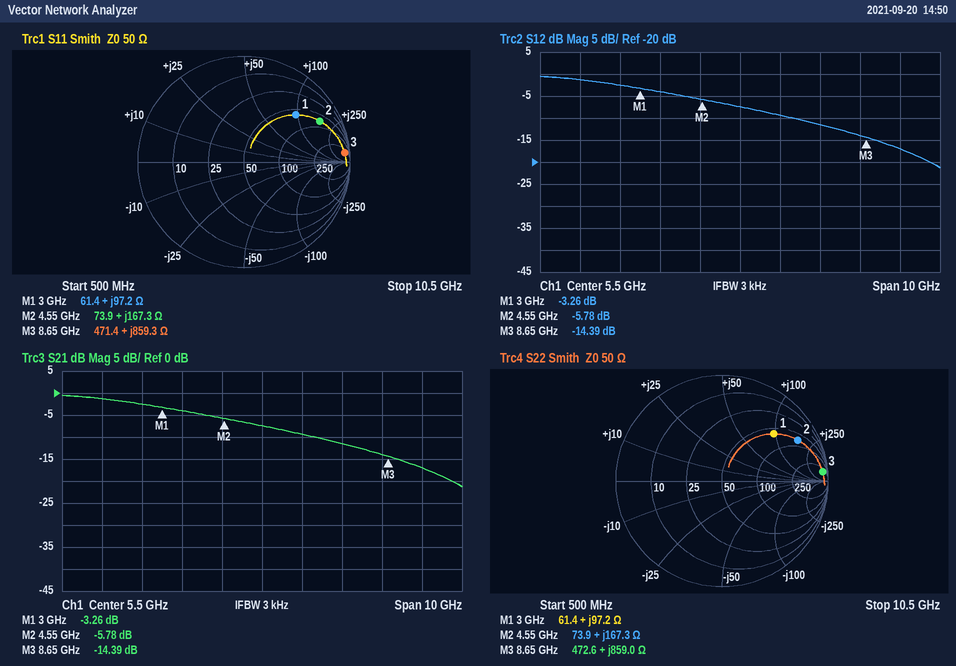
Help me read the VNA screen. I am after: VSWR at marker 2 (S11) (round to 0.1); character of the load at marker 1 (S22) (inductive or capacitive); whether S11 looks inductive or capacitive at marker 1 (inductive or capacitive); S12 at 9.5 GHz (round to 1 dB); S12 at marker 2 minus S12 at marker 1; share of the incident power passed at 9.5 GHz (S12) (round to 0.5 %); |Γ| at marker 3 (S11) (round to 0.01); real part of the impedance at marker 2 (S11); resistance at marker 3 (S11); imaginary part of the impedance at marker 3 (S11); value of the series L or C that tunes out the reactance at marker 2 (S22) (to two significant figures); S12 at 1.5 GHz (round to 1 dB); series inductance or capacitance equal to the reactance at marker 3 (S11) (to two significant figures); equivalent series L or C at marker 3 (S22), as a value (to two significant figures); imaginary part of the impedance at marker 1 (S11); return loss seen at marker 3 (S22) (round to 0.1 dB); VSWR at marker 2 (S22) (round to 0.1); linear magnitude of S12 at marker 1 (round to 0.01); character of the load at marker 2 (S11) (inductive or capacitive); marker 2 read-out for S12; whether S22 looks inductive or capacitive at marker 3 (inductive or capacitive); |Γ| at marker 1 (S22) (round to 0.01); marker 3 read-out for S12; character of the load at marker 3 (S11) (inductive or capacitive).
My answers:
9.6
inductive
inductive
-17 dB
-2.52 dB
2.0 %
0.95
73.9 Ω
471.4 Ω
+859.3 Ω
210 fF
-1 dB
16 nH
16 nH
+97.2 Ω
0.4 dB
9.6
0.69
inductive
-5.78 dB
inductive
0.66
-14.39 dB
inductive
